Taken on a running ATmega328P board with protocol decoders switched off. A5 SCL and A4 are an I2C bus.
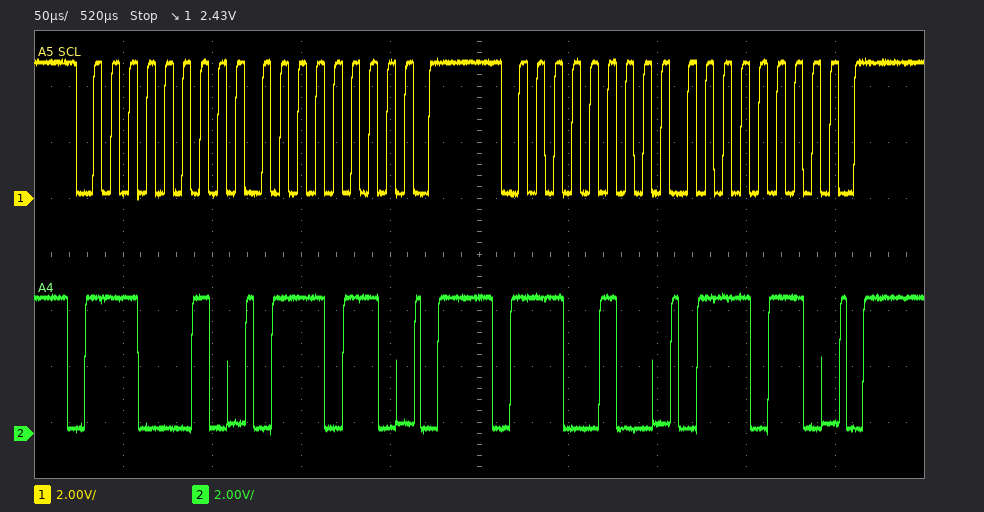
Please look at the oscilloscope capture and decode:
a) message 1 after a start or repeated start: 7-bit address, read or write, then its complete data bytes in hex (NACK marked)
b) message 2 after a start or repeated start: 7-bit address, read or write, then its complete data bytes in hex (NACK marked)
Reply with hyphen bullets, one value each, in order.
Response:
- 0x71 write: 76
- 0x72 write: 76
